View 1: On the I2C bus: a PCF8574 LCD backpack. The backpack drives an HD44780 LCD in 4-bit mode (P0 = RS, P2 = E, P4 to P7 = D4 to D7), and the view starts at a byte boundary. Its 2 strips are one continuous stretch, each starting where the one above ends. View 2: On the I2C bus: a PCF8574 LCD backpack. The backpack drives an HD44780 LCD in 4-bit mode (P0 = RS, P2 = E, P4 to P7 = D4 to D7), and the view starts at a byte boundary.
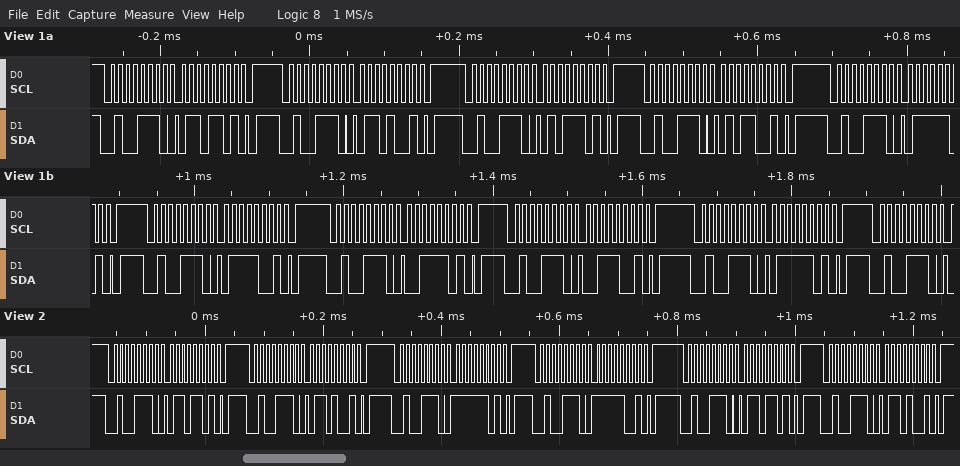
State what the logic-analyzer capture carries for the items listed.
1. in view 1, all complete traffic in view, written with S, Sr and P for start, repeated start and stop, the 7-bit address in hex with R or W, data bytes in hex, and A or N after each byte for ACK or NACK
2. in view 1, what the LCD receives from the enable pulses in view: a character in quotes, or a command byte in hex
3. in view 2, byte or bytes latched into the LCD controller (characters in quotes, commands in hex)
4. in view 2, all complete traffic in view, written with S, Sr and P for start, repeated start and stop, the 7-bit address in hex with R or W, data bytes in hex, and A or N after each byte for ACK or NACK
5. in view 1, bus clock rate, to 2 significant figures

S 27W A 6D A P S 27W A 69 A P S 27W A 5D A P S 27W A 59 A P S 27W A 7D A P S 27W A 79 A P S 27W A 3D A P S 27W A 39 A P S 27W A 7D A P S 27W A
'e' 's'
'o'
S 27W A 6D A P S 27W A 69 A P S 27W A FD A P S 27W A F9 A P S 27W A 6D A P S 27W A 69 A P
100 kHz
